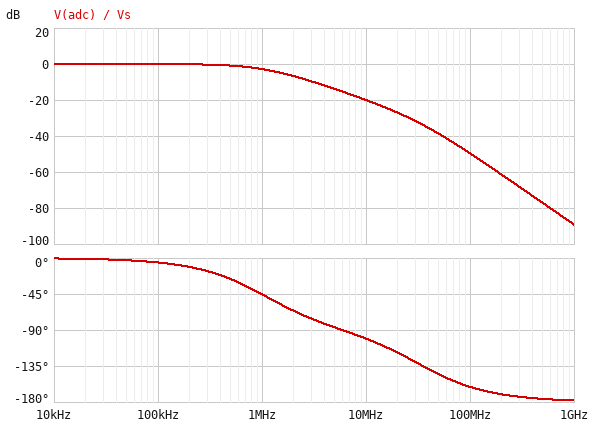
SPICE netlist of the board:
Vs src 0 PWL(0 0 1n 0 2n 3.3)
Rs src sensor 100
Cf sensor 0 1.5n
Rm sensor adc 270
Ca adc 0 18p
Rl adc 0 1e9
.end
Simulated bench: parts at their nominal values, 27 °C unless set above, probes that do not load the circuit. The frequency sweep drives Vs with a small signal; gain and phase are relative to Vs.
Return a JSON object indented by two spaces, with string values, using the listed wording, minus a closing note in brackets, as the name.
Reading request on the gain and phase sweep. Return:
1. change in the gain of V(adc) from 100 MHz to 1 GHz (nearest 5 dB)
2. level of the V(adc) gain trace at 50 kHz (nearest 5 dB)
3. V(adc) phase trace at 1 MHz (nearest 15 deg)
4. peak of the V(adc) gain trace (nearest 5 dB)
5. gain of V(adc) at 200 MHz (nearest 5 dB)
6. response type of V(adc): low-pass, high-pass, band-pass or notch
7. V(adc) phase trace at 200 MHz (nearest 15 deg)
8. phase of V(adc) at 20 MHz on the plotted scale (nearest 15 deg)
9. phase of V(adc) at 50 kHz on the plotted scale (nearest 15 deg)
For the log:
{
  "change in the gain of V(adc) from 100 MHz to 1 GHz": "-40 dB",
  "level of the V(adc) gain trace at 50 kHz": "0 dB",
  "V(adc) phase trace at 1 MHz": "-45 deg",
  "peak of the V(adc) gain trace": "0 dB",
  "gain of V(adc) at 200 MHz": "-60 dB",
  "response type of V(adc): low-pass, high-pass, band-pass or notch": "low-pass",
  "V(adc) phase trace at 200 MHz": "-165 deg",
  "phase of V(adc) at 20 MHz on the plotted scale": "-120 deg",
  "phase of V(adc) at 50 kHz on the plotted scale": "0 deg"
}
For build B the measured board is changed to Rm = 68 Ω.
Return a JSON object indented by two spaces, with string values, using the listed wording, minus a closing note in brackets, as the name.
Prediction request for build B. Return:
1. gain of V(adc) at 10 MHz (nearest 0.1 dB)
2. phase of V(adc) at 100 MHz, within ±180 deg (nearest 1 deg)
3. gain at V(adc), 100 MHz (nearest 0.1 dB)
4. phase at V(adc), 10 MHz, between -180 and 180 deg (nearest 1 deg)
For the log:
{
  "gain of V(adc) at 10 MHz": "-19.7 dB",
  "phase of V(adc) at 100 MHz, within ±180 deg": "-127 deg",
  "gain at V(adc), 100 MHz": "-41.6 dB",
  "phase at V(adc), 10 MHz, between -180 and 180 deg": "-88 deg"
}
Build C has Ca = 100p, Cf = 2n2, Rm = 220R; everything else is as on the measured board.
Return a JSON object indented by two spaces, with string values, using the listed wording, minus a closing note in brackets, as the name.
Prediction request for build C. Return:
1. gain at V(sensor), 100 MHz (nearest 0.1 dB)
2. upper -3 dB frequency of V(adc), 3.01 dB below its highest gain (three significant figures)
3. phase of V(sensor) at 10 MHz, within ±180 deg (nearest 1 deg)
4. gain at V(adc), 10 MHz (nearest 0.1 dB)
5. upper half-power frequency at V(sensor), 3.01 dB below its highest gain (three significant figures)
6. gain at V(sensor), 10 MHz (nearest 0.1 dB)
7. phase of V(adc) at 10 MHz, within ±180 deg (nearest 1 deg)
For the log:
{
  "gain at V(sensor), 100 MHz": "-42.8 dB",
  "upper -3 dB frequency of V(adc), 3.01 dB below its highest gain": "683 kHz",
  "phase of V(sensor) at 10 MHz, within ±180 deg": "-85 deg",
  "gain at V(adc), 10 MHz": "-27.6 dB",
  "upper half-power frequency at V(sensor), 3.01 dB below its highest gain": "689 kHz",
  "gain at V(sensor), 10 MHz": "-23.0 dB",
  "phase of V(adc) at 10 MHz, within ±180 deg": "-139 deg"
}
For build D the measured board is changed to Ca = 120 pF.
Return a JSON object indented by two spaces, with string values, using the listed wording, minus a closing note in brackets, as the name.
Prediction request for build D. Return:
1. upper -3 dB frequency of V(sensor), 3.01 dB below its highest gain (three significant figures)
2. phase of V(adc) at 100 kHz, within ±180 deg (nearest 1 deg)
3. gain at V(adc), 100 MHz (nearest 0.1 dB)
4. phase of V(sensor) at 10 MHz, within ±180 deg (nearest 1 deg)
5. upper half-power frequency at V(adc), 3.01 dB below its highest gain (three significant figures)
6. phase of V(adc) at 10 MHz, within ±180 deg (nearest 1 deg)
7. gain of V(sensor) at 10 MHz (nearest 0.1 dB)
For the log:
{
  "upper -3 dB frequency of V(sensor), 3.01 dB below its highest gain": "971 kHz",
  "phase of V(adc) at 100 kHz, within ±180 deg": "-7 deg",
  "gain at V(adc), 100 MHz": "-65.7 dB",
  "phase of V(sensor) at 10 MHz, within ±180 deg": "-82 deg",
  "upper half-power frequency at V(adc), 3.01 dB below its highest gain": "936 kHz",
  "phase of V(adc) at 10 MHz, within ±180 deg": "-146 deg",
  "gain of V(sensor) at 10 MHz": "-19.7 dB"
}
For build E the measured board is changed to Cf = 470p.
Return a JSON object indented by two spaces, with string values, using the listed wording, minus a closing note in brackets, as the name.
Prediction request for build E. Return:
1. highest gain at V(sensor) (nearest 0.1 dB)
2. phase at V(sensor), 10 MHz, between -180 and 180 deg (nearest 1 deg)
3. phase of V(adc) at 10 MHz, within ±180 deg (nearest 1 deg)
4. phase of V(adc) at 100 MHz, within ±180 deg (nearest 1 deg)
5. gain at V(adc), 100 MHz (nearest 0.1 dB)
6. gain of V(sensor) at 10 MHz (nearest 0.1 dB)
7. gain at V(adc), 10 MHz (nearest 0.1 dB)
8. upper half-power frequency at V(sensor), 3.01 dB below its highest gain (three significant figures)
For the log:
{
  "highest gain at V(sensor)": "0 dB",
  "phase at V(sensor), 10 MHz, between -180 and 180 deg": "-71 deg",
  "phase of V(adc) at 10 MHz, within ±180 deg": "-88 deg",
  "phase of V(adc) at 100 MHz, within ±180 deg": "-159 deg",
  "gain at V(adc), 100 MHz": "-39.6 dB",
  "gain of V(sensor) at 10 MHz": "-10.2 dB",
  "gain at V(adc), 10 MHz": "-10.6 dB",
  "upper half-power frequency at V(sensor), 3.01 dB below its highest gain": "3.25 MHz"
}
